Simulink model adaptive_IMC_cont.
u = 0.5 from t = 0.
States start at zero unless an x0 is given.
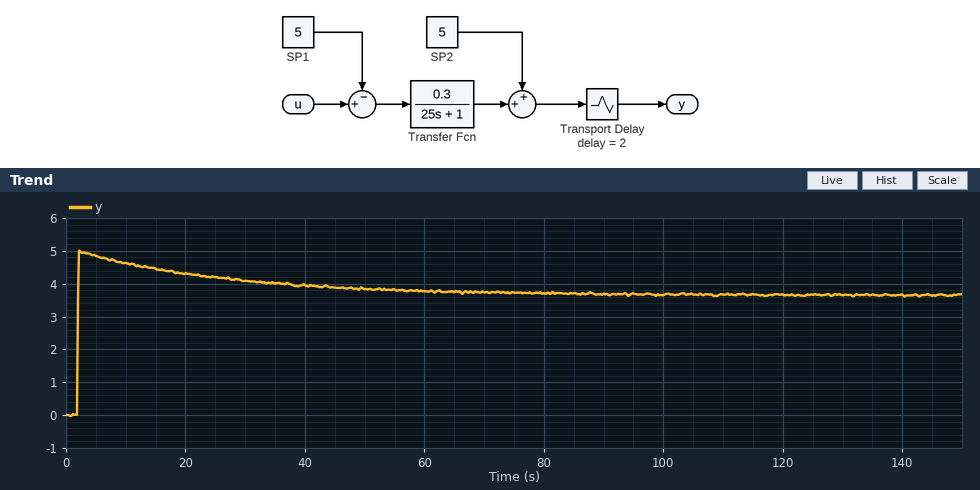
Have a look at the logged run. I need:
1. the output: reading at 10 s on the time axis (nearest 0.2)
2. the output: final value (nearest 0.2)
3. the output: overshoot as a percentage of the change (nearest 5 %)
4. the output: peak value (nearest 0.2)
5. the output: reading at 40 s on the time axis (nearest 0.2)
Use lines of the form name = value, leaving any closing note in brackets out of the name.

the output: reading at 10 s on the time axis = 4.6
the output: final value = 3.6
the output: overshoot as a percentage of the change = 35 %
the output: peak value = 5.0
the output: reading at 40 s on the time axis = 4.0
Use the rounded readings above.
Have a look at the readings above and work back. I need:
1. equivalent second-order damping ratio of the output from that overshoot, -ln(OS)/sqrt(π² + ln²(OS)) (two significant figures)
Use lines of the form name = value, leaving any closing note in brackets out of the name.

equivalent second-order damping ratio of the output from that overshoot, -ln(OS)/sqrt(π² + ln²(OS)) = 0.32
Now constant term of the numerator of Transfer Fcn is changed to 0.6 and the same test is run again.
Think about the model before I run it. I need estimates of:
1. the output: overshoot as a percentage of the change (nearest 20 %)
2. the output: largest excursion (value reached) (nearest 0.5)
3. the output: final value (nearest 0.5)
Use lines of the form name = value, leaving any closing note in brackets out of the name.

the output: overshoot as a percentage of the change = 120 %
the output: largest excursion (value reached) = 5.0
the output: final value = 2.5
